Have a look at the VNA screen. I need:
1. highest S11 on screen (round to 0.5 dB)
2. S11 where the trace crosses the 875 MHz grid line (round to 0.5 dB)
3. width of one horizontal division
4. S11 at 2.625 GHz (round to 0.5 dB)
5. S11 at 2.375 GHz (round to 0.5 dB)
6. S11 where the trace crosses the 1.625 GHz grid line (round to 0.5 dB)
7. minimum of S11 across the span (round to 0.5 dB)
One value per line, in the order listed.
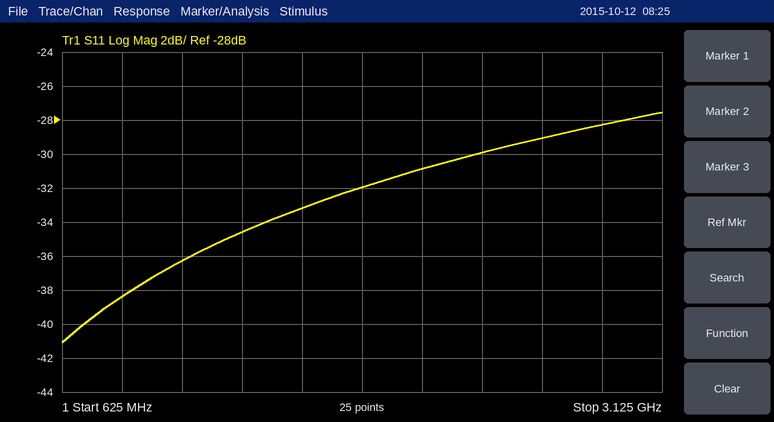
-27.5 dB
-38.5 dB
250 MHz
-29.0 dB
-30.0 dB
-33.0 dB
-41.0 dB
